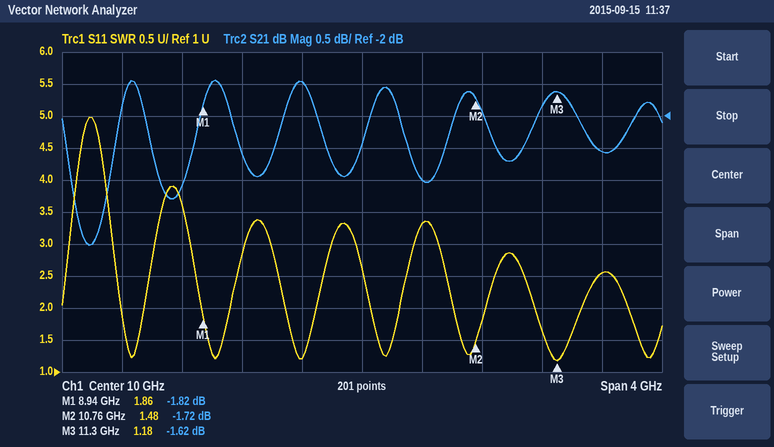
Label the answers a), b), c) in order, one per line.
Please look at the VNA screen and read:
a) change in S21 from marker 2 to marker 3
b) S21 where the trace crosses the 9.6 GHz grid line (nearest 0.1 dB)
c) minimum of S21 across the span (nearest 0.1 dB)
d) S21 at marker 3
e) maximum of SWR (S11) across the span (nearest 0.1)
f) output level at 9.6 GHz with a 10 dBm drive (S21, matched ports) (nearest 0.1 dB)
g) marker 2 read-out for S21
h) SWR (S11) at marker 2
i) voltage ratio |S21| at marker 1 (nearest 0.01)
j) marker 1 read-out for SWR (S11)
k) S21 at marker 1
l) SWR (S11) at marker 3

a) 0.10 dB
b) -1.5 dB
c) -4.0 dB
d) -1.62 dB
e) 5.0
f) 8.5 dBm
g) -1.72 dB
h) 1.48
i) 0.81
j) 1.86
k) -1.82 dB
l) 1.18
